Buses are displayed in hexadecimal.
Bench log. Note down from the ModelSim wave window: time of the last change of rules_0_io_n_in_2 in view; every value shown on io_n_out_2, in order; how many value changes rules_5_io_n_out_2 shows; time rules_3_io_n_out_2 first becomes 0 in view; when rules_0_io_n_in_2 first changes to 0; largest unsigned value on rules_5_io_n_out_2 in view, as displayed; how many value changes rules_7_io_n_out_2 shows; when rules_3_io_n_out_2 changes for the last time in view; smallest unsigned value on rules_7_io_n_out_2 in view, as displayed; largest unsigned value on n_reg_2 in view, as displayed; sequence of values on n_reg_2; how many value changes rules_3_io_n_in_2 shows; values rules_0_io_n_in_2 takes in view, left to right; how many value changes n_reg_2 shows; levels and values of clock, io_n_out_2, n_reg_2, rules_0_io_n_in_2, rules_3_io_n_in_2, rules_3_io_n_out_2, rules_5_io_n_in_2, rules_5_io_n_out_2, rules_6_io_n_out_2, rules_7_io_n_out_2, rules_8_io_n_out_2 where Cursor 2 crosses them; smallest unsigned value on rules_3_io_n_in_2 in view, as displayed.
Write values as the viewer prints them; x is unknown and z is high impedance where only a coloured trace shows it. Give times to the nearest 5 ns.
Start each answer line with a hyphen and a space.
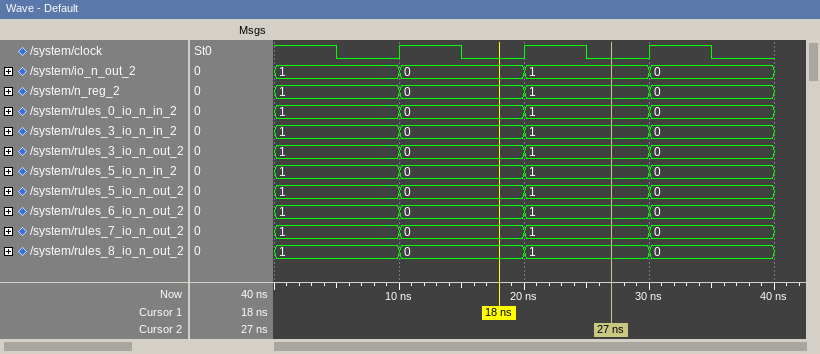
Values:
- 30 ns
- 1, 0, 1, 0
- 3
- 10 ns
- 10 ns
- 1
- 3
- 30 ns
- 0
- 1
- 1, 0, 1, 0
- 3
- 1, 0, 1, 0
- 3
- clock=0, io_n_out_2=1, n_reg_2=1, rules_0_io_n_in_2=1, rules_3_io_n_in_2=1, rules_3_io_n_out_2=1, rules_5_io_n_in_2=1, rules_5_io_n_out_2=1, rules_6_io_n_out_2=1, rules_7_io_n_out_2=1, rules_8_io_n_out_2=1
- 0
